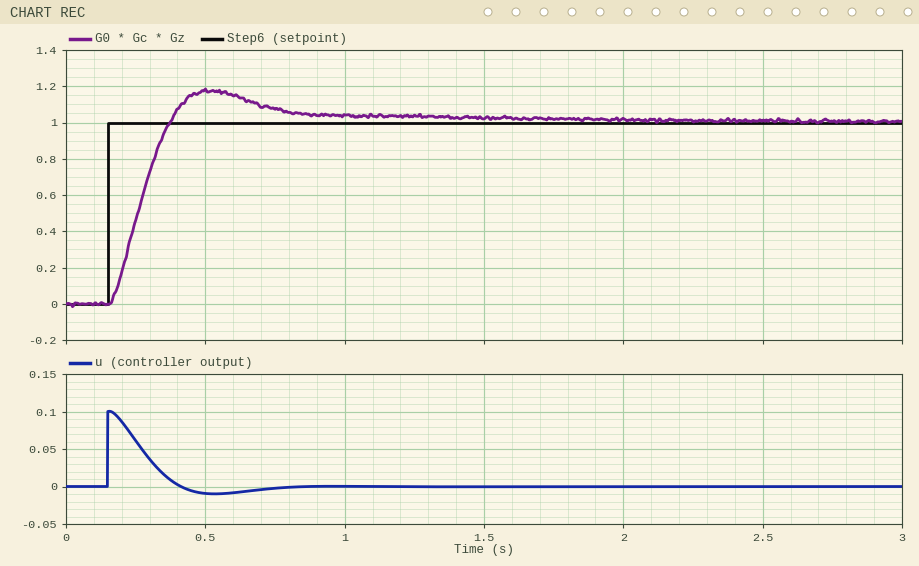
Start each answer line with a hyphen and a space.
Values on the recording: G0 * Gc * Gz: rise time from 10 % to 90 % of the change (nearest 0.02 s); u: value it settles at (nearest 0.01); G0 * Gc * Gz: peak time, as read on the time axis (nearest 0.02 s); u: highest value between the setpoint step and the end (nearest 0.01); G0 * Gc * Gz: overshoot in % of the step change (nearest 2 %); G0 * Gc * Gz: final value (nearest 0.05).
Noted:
- 0.16 s
- 0.00
- 0.52 s
- 0.10
- 18 %
- 1.00
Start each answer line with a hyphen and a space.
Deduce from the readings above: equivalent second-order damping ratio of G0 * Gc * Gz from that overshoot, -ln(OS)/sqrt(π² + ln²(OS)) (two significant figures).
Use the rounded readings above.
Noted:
- 0.48
